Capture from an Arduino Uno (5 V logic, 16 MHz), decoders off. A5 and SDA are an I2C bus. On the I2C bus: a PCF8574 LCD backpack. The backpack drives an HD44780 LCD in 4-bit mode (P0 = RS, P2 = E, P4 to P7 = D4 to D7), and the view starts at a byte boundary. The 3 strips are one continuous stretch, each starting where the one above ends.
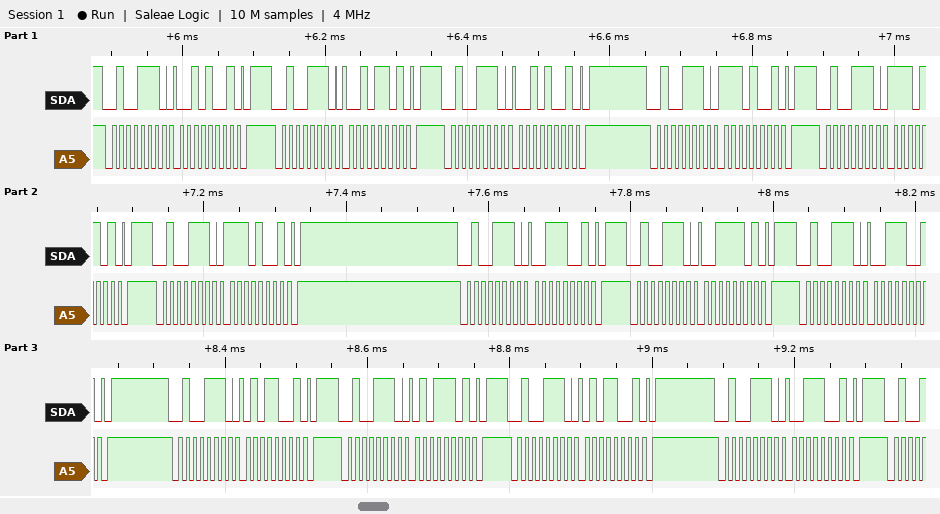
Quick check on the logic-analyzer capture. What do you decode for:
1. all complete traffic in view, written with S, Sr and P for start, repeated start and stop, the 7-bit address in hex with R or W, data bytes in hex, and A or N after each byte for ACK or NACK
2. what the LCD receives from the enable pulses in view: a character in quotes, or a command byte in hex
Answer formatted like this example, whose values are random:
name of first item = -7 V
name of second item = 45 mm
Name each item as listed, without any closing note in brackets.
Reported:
all complete traffic in view, written with S, Sr and P for start, repeated start and stop, the 7-bit address in hex with R or W, data bytes in hex, and A or N after each byte for ACK or NACK = S 27W A 29 A P S 27W A 2D A P S 27W A 29 A P S 27W A E9 A P S 27W A ED A P S 27W A E9 A P S 27W A 39 A P S 27W A 3D A P S 27W A 39 A P S 27W A 59 A P S 27W A 5D A P S 27W A 59 A P S 27W A 39 A P
what the LCD receives from the enable pulses in view: a character in quotes, or a command byte in hex = '.' '5'
